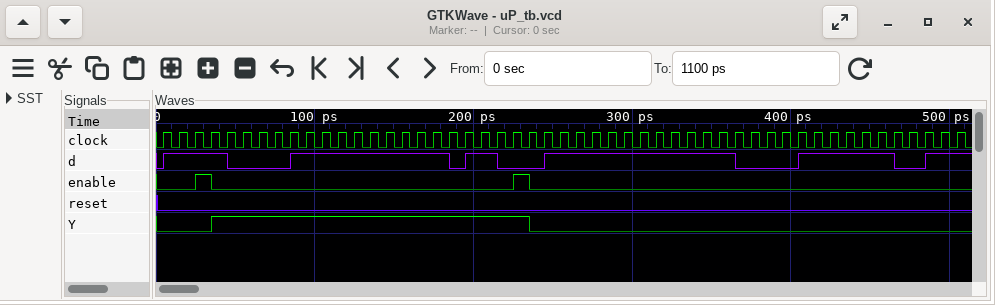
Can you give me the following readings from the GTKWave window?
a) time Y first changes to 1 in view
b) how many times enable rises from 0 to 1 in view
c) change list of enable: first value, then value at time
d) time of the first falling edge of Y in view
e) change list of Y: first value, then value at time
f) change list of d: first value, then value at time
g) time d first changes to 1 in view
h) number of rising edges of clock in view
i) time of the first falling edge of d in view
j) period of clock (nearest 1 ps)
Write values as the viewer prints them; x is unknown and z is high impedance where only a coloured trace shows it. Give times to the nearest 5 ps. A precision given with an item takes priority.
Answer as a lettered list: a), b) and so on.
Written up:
a) 35 ps
b) 2
c) 0, 1 at 25 ps, 0 at 35 ps, 1 at 225 ps, 0 at 235 ps
d) 235 ps
e) 0, 1 at 35 ps, 0 at 235 ps
f) 0, 1 at 5 ps, 0 at 45 ps, 1 at 85 ps, 0 at 185 ps, 1 at 195 ps, 0 at 215 ps, 1 at 245 ps, 0 at 365 ps, 1 at 405 ps, 0 at 465 ps, 1 at 485 ps
g) 5 ps
h) 51
i) 45 ps
j) 10 ps
